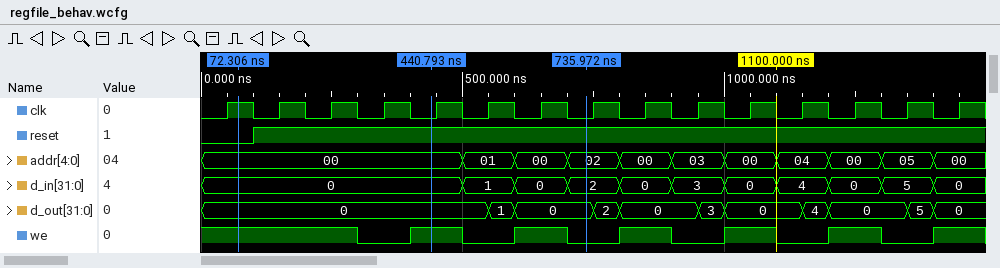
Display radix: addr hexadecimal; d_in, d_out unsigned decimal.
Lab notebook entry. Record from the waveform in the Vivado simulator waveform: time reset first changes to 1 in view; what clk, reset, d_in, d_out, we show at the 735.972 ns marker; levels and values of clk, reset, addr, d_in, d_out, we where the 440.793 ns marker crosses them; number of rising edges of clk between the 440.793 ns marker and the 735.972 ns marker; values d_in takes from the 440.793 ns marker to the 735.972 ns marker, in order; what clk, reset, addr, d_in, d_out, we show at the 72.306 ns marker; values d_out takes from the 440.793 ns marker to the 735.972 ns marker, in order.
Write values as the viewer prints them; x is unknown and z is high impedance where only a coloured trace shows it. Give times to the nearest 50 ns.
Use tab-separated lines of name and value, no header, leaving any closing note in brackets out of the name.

time reset first changes to 1 in view	100 ns
what clk, reset, d_in, d_out, we show at the 735.972 ns marker	clk=0, reset=1, d_in=2, d_out=0, we=0
levels and values of clk, reset, addr, d_in, d_out, we where the 440.793 ns marker crosses them	clk=0, reset=1, addr=00, d_in=0, d_out=0, we=1
number of rising edges of clk between the 440.793 ns marker and the 735.972 ns marker	3
values d_in takes from the 440.793 ns marker to the 735.972 ns marker, in order	0, 1, 0, 2
what clk, reset, addr, d_in, d_out, we show at the 72.306 ns marker	clk=1, reset=0, addr=00, d_in=0, d_out=0, we=1
values d_out takes from the 440.793 ns marker to the 735.972 ns marker, in order	0, 1, 0
